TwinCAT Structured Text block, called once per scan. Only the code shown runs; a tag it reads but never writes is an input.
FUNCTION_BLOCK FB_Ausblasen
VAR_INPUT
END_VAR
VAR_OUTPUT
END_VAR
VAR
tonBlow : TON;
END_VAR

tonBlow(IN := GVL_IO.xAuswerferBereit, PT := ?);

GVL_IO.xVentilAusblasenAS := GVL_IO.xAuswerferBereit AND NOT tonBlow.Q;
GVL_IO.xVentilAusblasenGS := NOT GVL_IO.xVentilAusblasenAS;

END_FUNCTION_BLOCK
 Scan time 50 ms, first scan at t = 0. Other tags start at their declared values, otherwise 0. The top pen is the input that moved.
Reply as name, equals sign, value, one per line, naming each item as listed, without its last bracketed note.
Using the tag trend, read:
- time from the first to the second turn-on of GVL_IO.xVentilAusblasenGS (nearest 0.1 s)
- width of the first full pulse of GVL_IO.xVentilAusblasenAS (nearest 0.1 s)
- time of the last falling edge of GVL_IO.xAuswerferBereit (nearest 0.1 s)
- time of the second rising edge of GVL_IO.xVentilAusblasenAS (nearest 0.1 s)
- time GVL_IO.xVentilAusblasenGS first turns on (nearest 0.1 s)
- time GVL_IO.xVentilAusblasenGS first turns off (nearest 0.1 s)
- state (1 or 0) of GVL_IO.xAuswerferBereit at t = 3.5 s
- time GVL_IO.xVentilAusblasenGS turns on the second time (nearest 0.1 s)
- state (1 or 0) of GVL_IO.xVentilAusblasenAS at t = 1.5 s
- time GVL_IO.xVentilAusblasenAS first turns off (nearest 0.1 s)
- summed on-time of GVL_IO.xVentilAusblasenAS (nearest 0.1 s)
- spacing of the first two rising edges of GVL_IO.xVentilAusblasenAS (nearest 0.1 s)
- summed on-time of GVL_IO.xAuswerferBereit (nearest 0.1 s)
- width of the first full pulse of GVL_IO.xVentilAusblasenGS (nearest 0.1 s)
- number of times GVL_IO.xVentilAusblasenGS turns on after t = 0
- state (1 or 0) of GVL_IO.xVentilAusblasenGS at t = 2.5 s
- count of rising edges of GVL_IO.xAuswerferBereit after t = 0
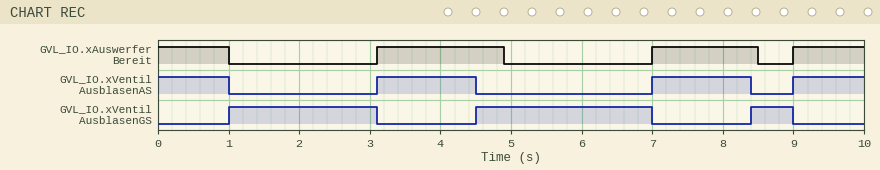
time from the first to the second turn-on of GVL_IO.xVentilAusblasenGS = 3.5 s
width of the first full pulse of GVL_IO.xVentilAusblasenAS = 1.4 s
time of the last falling edge of GVL_IO.xAuswerferBereit = 8.5 s
time of the second rising edge of GVL_IO.xVentilAusblasenAS = 7.0 s
time GVL_IO.xVentilAusblasenGS first turns on = 1.0 s
time GVL_IO.xVentilAusblasenGS first turns off = 3.1 s
state (1 or 0) of GVL_IO.xAuswerferBereit at t = 3.5 s = 1
time GVL_IO.xVentilAusblasenGS turns on the second time = 4.5 s
state (1 or 0) of GVL_IO.xVentilAusblasenAS at t = 1.5 s = 0
time GVL_IO.xVentilAusblasenAS first turns off = 1.0 s
summed on-time of GVL_IO.xVentilAusblasenAS = 4.8 s
spacing of the first two rising edges of GVL_IO.xVentilAusblasenAS = 3.9 s
summed on-time of GVL_IO.xAuswerferBereit = 5.3 s
width of the first full pulse of GVL_IO.xVentilAusblasenGS = 2.1 s
number of times GVL_IO.xVentilAusblasenGS turns on after t = 0 = 3
state (1 or 0) of GVL_IO.xVentilAusblasenGS at t = 2.5 s = 1
count of rising edges of GVL_IO.xAuswerferBereit after t = 0 = 3
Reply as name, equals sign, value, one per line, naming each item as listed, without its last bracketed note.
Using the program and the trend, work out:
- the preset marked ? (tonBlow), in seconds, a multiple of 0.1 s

the preset marked ? (tonBlow), in seconds, a multiple of 0.1 s = 1.4 s
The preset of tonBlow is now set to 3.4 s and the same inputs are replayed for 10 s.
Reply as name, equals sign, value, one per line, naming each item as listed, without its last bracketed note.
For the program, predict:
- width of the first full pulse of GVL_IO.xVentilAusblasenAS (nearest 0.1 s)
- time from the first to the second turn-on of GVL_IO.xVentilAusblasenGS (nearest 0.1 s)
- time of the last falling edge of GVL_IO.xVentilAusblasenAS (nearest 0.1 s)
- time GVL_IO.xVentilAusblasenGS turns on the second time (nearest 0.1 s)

width of the first full pulse of GVL_IO.xVentilAusblasenAS = 1.8 s
time from the first to the second turn-on of GVL_IO.xVentilAusblasenGS = 3.9 s
time of the last falling edge of GVL_IO.xVentilAusblasenAS = 8.5 s
time GVL_IO.xVentilAusblasenGS turns on the second time = 4.9 s
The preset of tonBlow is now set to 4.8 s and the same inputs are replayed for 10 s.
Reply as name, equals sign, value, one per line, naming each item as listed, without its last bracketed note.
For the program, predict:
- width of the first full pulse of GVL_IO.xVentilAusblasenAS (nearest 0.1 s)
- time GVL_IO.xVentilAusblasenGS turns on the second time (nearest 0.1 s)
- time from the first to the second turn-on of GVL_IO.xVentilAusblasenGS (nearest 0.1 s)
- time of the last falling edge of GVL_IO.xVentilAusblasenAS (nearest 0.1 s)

width of the first full pulse of GVL_IO.xVentilAusblasenAS = 1.8 s
time GVL_IO.xVentilAusblasenGS turns on the second time = 4.9 s
time from the first to the second turn-on of GVL_IO.xVentilAusblasenGS = 3.9 s
time of the last falling edge of GVL_IO.xVentilAusblasenAS = 8.5 s
